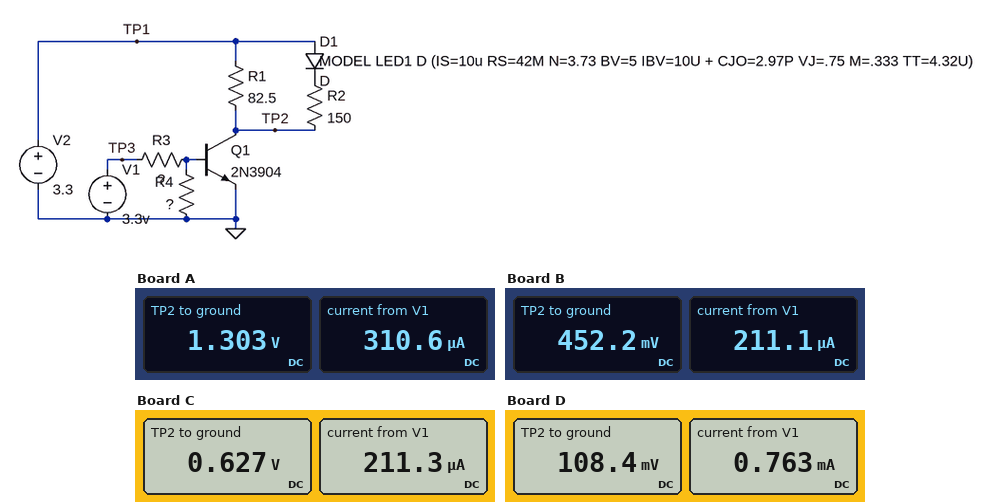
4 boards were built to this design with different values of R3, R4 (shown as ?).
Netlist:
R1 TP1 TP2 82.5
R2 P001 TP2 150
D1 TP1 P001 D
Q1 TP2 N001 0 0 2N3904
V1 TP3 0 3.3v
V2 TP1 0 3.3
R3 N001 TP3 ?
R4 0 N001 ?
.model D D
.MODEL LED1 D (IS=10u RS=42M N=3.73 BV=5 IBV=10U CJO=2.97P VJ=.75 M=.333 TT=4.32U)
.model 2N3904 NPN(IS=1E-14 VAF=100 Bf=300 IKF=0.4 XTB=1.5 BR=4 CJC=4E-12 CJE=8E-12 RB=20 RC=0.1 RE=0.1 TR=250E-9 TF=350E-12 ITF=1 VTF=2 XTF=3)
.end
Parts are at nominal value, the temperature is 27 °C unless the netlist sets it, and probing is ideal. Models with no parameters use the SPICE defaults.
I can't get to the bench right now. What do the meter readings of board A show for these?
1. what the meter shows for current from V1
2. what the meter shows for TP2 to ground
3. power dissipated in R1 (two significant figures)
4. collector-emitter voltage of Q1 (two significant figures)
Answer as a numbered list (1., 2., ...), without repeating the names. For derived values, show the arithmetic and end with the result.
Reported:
1. 310.6 µA
2. 1.303 V
3. (3.3 V - 1.303 V)^2 / 82.5 Ω = 48 mW
4. 1.303 V = 1.3 V
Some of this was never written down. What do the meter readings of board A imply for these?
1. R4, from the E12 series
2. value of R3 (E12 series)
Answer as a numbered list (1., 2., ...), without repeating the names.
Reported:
1. 3.9 kΩ
2. 8.2 kΩ
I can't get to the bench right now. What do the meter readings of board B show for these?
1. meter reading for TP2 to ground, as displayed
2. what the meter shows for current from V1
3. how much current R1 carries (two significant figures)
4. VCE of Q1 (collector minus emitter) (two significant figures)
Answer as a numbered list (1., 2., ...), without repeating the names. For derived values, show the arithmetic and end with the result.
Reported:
1. 452.2 mV
2. 211.1 µA
3. (3.3 V - 452.2 mV) / 82.5 Ω = 35 mA
4. 452.2 mV = 450 mV
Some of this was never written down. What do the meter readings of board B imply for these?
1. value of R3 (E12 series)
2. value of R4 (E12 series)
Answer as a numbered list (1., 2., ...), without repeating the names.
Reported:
1. 12 kΩ
2. 27 kΩ
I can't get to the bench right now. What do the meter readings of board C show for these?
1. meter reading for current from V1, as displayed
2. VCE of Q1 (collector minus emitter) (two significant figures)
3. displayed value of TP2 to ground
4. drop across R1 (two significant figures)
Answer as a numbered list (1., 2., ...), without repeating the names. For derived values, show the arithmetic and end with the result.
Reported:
1. 211.3 µA
2. 627 mV = 630 mV
3. 0.627 V
4. 3.3 V - 627 mV = 2.7 V
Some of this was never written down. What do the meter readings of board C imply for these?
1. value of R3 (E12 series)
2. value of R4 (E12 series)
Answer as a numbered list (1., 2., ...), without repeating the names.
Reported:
1. 12 kΩ
2. 18 kΩ
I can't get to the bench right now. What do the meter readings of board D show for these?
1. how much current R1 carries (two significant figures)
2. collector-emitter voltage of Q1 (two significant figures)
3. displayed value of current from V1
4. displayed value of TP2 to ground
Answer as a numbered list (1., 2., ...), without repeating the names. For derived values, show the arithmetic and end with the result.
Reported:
1. (3.3 V - 108.4 mV) / 82.5 Ω = 39 mA
2. 108.4 mV = 110 mV
3. 0.763 mA
4. 108.4 mV
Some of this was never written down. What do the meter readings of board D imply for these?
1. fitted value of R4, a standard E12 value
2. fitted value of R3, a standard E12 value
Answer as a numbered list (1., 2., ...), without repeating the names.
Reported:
1. 4.7 kΩ
2. 3.3 kΩ
